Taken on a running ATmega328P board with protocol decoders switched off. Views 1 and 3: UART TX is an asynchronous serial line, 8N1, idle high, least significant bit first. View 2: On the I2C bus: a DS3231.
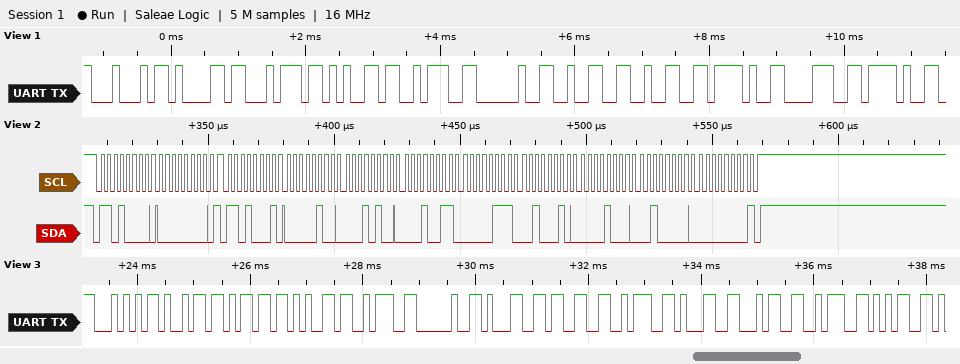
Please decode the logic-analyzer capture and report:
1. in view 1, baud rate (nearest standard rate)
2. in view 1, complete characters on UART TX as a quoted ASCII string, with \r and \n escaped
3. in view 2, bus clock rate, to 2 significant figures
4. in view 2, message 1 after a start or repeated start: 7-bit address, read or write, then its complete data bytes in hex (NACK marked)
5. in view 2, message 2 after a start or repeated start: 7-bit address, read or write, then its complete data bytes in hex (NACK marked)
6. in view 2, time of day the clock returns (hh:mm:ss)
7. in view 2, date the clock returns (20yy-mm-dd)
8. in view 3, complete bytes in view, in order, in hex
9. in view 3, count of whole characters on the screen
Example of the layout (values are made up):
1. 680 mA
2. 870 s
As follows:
1. 9600 baud
2. "Date: 22/8/"
3. 400 kHz
4. 0x68 write: 00
5. 0x68 read: 04 14 13 07 22 08 20 00 NACK
6. 13:14:04
7. 2020-08-22
8. 54 69 6D 65 3A 20 31 33 3A 31 34 3A 35
9. 13
